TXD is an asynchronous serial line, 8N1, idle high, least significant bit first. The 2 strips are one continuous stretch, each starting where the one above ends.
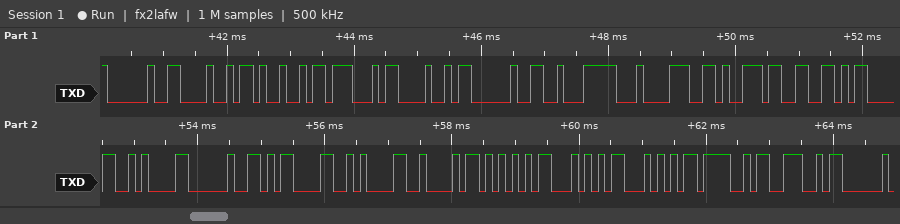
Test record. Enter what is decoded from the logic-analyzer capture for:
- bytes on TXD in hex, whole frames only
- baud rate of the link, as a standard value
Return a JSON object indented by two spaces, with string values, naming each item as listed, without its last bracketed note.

{
  "bytes on TXD in hex, whole frames only": "0x20 0x48 0x49 0x47 0x48 0x20 0xE2 0x84 0x96 0x33 0x0D 0x0A 0x20 0x0D 0x0A 0x42 0x55 0x54 0x54 0x4F 0x4E",
  "baud rate of the link, as a standard value": "9600 baud"
}
